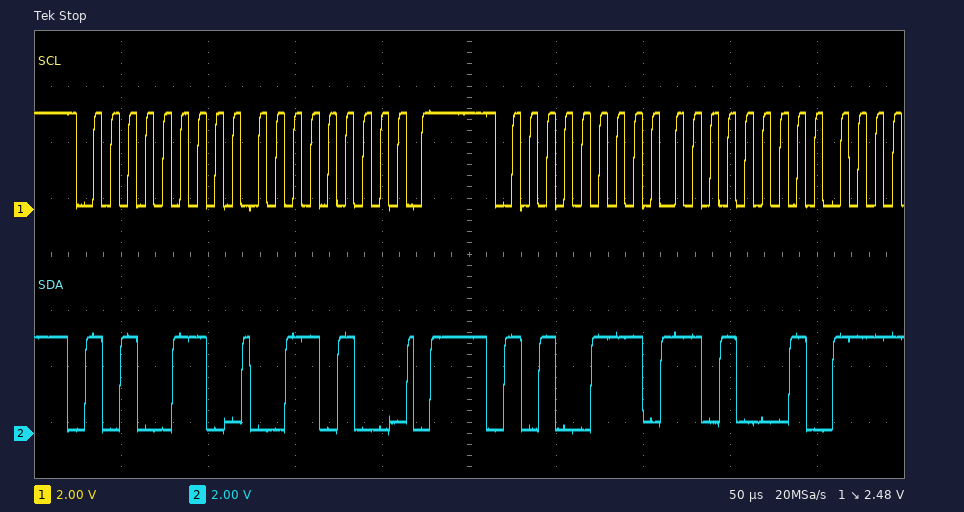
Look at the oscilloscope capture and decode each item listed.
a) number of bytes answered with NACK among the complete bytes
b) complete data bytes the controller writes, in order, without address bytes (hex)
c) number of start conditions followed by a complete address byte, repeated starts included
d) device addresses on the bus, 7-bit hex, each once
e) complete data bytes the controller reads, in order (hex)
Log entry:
0
34
2
0x53
D1
